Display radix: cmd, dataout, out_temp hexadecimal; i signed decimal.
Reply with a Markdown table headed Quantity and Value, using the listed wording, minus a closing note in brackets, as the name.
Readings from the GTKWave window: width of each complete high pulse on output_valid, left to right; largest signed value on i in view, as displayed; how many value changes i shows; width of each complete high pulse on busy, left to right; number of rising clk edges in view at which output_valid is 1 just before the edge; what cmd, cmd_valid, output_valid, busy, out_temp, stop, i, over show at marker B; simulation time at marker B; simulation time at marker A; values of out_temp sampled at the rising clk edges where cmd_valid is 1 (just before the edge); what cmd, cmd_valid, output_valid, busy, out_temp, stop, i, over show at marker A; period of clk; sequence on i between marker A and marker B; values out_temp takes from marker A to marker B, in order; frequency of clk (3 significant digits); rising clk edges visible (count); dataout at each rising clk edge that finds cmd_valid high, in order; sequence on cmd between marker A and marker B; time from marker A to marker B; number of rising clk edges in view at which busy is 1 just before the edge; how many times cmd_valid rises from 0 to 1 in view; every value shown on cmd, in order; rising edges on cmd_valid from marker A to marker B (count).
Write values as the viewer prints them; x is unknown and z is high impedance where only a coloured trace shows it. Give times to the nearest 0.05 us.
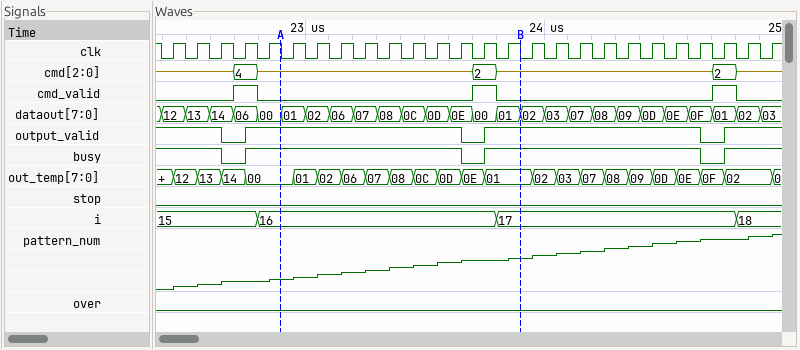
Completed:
| Quantity | Value |
|---|---|
| width of each complete high pulse on output_valid, left to right | 0.9 us, 0.9 us |
| largest signed value on i in view, as displayed | 18 |
| how many value changes i shows | 3 |
| width of each complete high pulse on busy, left to right | 0.9 us, 0.9 us |
| number of rising clk edges in view at which output_valid is 1 just before the edge | 23 |
| what cmd, cmd_valid, output_valid, busy, out_temp, stop, i, over show at marker B | cmd=z, cmd_valid=0, output_valid=1, busy=1, out_temp=01, stop=0, i=17, over=0 |
| simulation time at marker B | 23.9 us |
| simulation time at marker A | 22.9 us |
| values of out_temp sampled at the rising clk edges where cmd_valid is 1 | 14, 0E, 0F |
| what cmd, cmd_valid, output_valid, busy, out_temp, stop, i, over show at marker A | cmd=z, cmd_valid=0, output_valid=1, busy=1, out_temp=00, stop=0, i=16, over=0 |
| period of clk | 0.1 us |
| sequence on i between marker A and marker B | 16, 17 |
| values out_temp takes from marker A to marker B, in order | 00, 01, 02, 06, 07, 08, 0C, 0D, 0E, 01 |
| frequency of clk | 10.0 MHz |
| rising clk edges visible | 26 |
| dataout at each rising clk edge that finds cmd_valid high, in order | 06, 00, 01 |
| sequence on cmd between marker A and marker B | z, 2, z |
| time from marker A to marker B | 1 us |
| number of rising clk edges in view at which busy is 1 just before the edge | 23 |
| how many times cmd_valid rises from 0 to 1 in view | 3 |
| every value shown on cmd, in order | z, 4, z, 2, z, 2, z |
| rising edges on cmd_valid from marker A to marker B | 1 |
